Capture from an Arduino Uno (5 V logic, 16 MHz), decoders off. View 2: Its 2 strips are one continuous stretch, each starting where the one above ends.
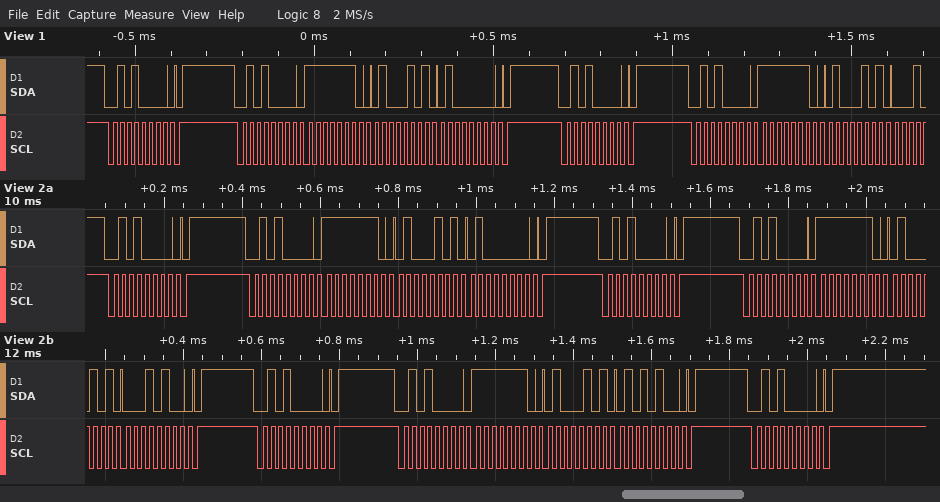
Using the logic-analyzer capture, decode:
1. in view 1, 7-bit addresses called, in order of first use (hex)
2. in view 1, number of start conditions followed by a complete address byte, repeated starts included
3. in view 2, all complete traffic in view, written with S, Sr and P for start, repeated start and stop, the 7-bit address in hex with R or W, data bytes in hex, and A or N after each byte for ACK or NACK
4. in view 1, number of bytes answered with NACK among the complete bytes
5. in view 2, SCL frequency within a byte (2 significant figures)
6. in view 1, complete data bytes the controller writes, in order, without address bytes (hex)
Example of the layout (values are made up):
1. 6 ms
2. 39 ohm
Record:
1. 0x28
2. 4
3. S 28W A P S 28W A FE A 45 A 40 A P S 28W A P S 28W A FE A 45 A 14 A P S 28W A P S 28W A FE A 45 A 54 A P S 28W A P
4. 0
5. 50 kHz
6. FE 45 40 FE 45
